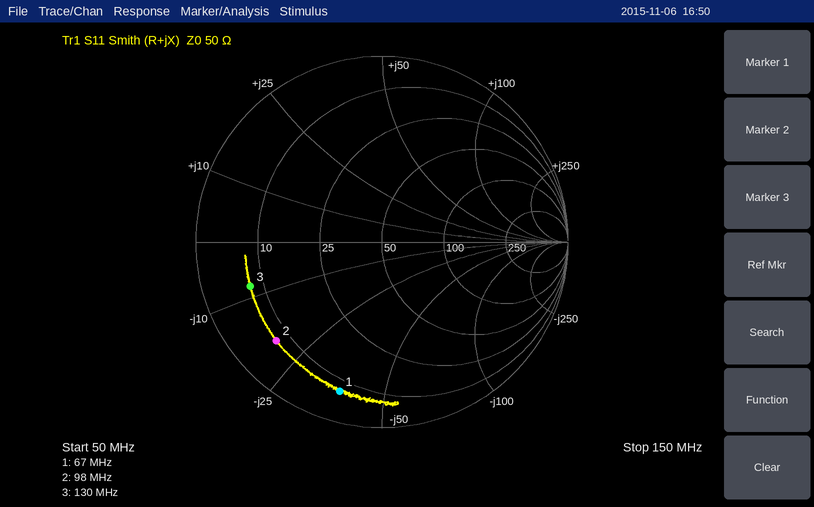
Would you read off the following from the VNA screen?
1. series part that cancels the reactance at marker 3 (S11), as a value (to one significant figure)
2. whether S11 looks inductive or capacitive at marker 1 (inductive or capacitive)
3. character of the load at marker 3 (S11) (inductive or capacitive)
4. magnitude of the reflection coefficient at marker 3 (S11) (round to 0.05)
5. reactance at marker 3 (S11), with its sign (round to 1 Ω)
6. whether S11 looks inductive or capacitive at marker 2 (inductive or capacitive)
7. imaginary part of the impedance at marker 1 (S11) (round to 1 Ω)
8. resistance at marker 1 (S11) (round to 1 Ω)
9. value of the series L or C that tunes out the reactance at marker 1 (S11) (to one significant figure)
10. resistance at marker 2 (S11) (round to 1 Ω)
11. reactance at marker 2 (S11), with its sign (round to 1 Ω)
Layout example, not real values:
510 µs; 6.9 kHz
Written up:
10 nH; capacitive; capacitive; 0.75; -8 Ω; capacitive; -37 Ω; 7 Ω; 90 nH; 7 Ω; -19 Ω
